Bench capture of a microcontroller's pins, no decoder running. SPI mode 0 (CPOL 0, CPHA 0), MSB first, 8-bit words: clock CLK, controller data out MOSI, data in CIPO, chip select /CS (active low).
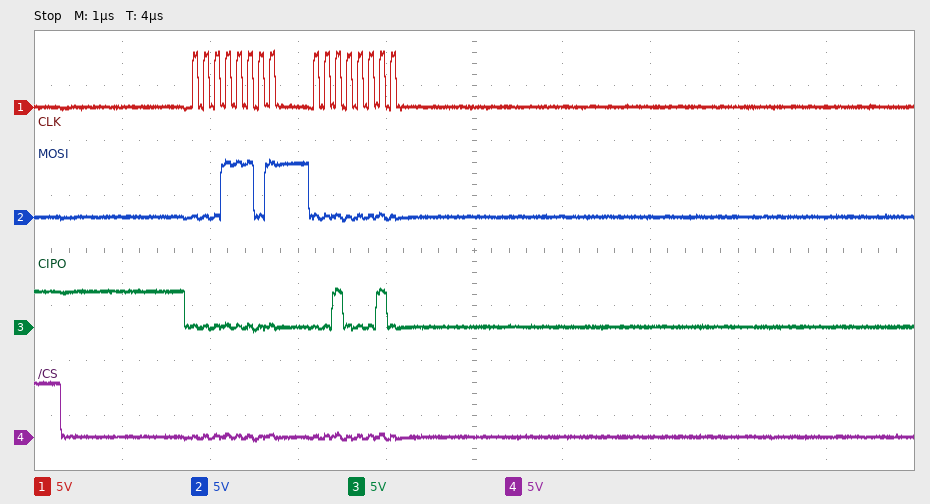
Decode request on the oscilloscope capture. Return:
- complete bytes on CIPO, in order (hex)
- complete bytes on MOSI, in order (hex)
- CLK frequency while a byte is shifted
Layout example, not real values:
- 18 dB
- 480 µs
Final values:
- 0x00 0x22
- 0x1D 0x00
- 8 MHz
